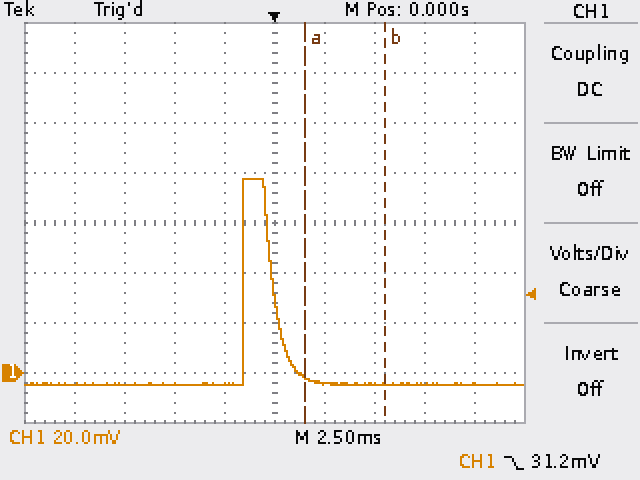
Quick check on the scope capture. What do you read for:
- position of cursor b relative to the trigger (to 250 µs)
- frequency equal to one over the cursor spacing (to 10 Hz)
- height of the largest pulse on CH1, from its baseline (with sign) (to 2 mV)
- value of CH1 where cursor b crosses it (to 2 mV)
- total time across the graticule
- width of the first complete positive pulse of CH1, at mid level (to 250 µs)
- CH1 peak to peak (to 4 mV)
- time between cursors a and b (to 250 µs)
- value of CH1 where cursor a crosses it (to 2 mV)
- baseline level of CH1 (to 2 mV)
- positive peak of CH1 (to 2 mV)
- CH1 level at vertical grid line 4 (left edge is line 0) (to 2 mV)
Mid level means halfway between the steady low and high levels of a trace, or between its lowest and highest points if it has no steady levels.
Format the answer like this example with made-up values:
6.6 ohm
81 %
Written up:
+5.50 ms
250 Hz
+82 mV
-4 mV
25 ms
1.50 ms
84 mV
4.00 ms
-2 mV
-4 mV
78 mV
-4 mV
